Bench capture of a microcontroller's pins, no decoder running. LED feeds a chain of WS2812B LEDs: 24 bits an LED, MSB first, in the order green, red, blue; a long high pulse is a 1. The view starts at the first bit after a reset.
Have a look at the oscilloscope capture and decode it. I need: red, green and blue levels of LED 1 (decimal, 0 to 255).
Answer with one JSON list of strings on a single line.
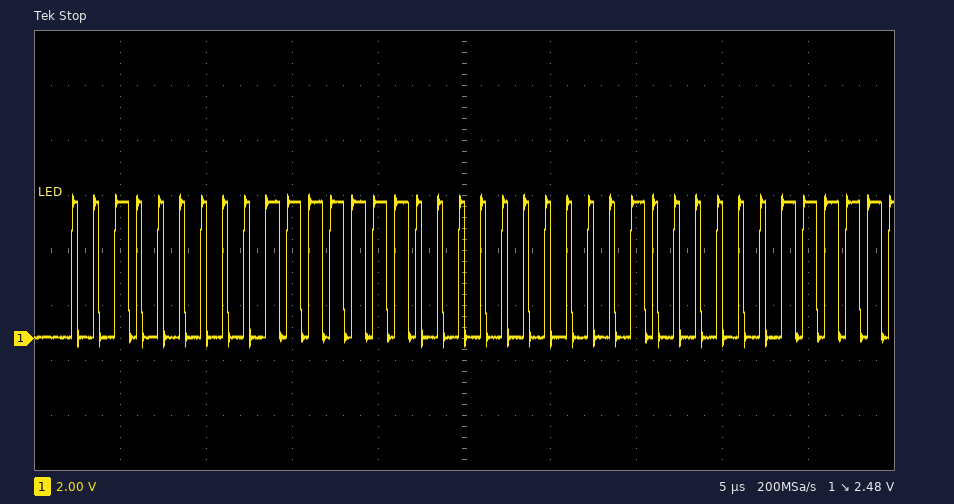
["127, 32, 0"]
